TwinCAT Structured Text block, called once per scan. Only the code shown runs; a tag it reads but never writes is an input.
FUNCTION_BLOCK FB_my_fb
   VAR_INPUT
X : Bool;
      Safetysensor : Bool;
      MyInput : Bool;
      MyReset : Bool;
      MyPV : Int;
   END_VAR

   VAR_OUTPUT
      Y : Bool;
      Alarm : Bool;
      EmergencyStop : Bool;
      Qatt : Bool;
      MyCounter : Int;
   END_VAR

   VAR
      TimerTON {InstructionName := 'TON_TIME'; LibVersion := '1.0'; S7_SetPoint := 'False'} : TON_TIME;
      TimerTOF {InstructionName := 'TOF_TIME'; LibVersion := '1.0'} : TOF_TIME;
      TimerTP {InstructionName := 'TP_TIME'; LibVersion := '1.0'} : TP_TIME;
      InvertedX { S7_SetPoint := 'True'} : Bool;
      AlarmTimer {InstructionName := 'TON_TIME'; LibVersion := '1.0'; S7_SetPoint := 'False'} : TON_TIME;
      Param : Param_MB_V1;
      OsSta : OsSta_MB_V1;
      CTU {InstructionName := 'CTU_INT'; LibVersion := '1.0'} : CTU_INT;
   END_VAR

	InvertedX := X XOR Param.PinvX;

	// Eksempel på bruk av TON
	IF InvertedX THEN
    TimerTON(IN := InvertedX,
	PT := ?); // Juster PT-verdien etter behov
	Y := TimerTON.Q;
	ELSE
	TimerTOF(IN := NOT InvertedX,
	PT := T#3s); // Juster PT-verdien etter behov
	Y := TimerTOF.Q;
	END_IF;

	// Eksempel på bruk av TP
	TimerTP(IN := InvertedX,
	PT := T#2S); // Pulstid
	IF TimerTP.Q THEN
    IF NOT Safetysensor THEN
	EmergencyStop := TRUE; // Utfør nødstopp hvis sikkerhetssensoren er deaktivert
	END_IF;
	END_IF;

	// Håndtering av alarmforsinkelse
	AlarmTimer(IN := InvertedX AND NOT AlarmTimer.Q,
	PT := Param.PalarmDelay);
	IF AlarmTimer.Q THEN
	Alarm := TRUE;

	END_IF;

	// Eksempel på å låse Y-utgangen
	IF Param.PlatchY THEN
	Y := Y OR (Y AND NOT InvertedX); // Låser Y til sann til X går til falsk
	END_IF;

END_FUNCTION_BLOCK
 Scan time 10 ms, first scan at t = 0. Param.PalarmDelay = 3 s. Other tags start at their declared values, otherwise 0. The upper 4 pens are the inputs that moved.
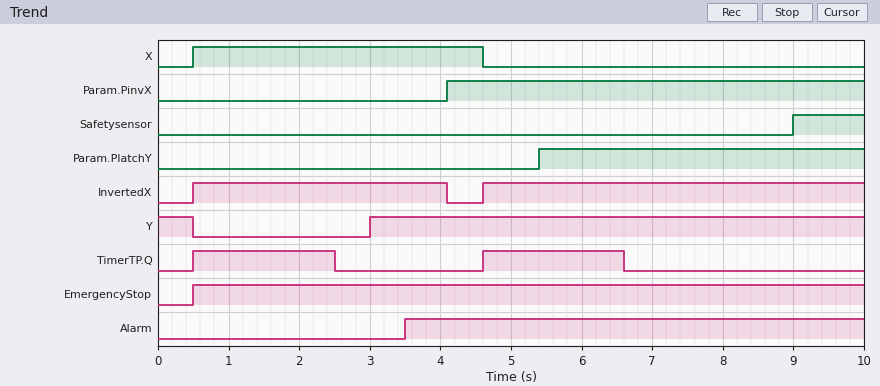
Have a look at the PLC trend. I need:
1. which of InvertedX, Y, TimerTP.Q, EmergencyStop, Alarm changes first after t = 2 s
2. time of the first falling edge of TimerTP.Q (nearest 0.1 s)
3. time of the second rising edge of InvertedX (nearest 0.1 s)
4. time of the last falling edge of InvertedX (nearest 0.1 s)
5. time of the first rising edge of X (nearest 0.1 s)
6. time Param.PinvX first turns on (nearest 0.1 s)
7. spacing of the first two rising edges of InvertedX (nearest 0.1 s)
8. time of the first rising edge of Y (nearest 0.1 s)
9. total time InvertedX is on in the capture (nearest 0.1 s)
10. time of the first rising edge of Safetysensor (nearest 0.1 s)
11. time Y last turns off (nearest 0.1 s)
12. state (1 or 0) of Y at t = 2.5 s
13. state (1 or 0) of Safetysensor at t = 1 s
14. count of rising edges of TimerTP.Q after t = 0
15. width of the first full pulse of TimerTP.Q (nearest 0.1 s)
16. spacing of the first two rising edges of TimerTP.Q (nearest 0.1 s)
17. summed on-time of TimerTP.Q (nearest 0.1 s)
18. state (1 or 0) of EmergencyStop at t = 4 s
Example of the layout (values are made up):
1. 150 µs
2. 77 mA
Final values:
1. TimerTP.Q
2. 2.5 s
3. 4.6 s
4. 4.1 s
5. 0.5 s
6. 4.1 s
7. 4.1 s
8. 3.0 s
9. 9.0 s
10. 9.0 s
11. 0.5 s
12. 0
13. 0
14. 2
15. 2.0 s
16. 4.1 s
17. 4.0 s
18. 1
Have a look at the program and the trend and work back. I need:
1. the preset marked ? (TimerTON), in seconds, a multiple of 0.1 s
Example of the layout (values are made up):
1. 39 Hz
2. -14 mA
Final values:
1. 2.5 s
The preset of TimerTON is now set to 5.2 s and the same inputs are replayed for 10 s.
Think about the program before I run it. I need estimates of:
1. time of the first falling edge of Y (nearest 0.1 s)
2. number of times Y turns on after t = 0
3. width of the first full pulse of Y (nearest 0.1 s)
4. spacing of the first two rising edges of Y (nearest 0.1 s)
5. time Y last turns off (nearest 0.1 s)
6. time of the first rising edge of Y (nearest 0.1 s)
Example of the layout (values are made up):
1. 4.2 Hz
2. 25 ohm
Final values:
1. 0.5 s
2. 2
3. 0.5 s
4. 1.6 s
5. 4.6 s
6. 4.1 s
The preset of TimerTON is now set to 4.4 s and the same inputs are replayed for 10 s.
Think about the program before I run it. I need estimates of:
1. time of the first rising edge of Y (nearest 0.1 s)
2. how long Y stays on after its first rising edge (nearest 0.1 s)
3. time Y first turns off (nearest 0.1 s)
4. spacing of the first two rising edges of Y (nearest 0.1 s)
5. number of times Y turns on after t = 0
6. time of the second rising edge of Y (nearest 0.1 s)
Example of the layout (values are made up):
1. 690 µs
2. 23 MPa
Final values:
1. 4.1 s
2. 0.5 s
3. 0.5 s
4. 0.8 s
5. 2
6. 4.9 s
